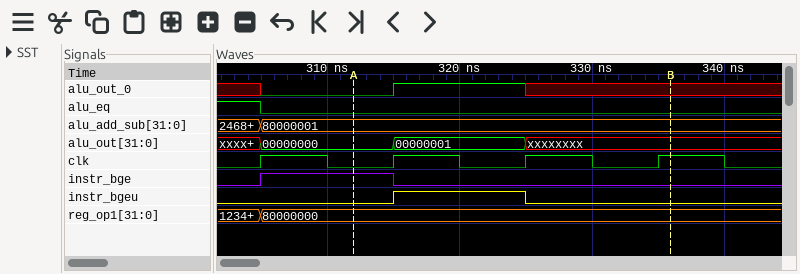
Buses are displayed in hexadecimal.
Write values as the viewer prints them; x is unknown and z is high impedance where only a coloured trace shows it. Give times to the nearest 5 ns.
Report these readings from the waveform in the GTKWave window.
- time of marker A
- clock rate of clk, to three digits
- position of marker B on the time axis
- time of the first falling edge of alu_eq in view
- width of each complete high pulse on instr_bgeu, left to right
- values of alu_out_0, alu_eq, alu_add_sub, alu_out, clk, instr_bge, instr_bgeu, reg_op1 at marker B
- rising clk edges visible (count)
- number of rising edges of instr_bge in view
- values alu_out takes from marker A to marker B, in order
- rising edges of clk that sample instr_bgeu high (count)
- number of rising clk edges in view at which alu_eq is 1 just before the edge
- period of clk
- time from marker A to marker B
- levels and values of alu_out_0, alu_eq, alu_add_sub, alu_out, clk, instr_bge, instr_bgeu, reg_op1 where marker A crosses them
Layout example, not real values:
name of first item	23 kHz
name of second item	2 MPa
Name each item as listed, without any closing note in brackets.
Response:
time of marker A	310 ns
clock rate of clk, to three digits	100 MHz
position of marker B on the time axis	335 ns
time of the first falling edge of alu_eq in view	305 ns
width of each complete high pulse on instr_bgeu, left to right	10 ns
values of alu_out_0, alu_eq, alu_add_sub, alu_out, clk, instr_bge, instr_bgeu, reg_op1 at marker B	alu_out_0=x, alu_eq=0, alu_add_sub=80000001, alu_out=xxxxxxxx, clk=1, instr_bge=0, instr_bgeu=0, reg_op1=80000000
rising clk edges visible	4
number of rising edges of instr_bge in view	1
values alu_out takes from marker A to marker B, in order	00000000, 00000001, xxxxxxxx
rising edges of clk that sample instr_bgeu high	1
number of rising clk edges in view at which alu_eq is 1 just before the edge	1
period of clk	10 ns
time from marker A to marker B	25 ns
levels and values of alu_out_0, alu_eq, alu_add_sub, alu_out, clk, instr_bge, instr_bgeu, reg_op1 where marker A crosses them	alu_out_0=0, alu_eq=0, alu_add_sub=80000001, alu_out=00000000, clk=0, instr_bge=1, instr_bgeu=0, reg_op1=80000000
